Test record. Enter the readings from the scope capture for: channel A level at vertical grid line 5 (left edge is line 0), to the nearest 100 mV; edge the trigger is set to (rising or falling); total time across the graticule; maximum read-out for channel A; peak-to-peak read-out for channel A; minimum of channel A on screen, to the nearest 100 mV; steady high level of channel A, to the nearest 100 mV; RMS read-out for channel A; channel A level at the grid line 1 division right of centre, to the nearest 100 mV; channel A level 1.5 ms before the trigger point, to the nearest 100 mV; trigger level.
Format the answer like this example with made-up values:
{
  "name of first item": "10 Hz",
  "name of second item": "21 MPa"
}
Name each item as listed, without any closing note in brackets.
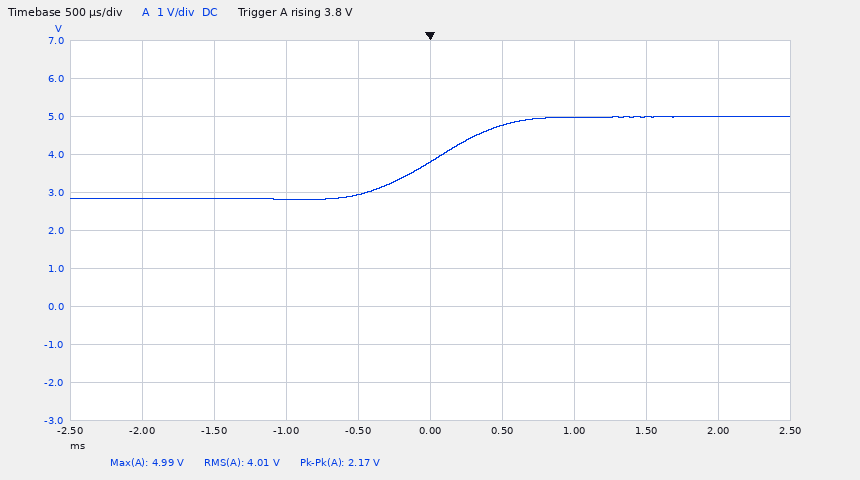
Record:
{
  "channel A level at vertical grid line 5 (left edge is line 0), to the nearest 100 mV": "3.8 V",
  "edge the trigger is set to": "rising",
  "total time across the graticule": "5 ms",
  "maximum read-out for channel A": "4.99 V",
  "peak-to-peak read-out for channel A": "2.17 V",
  "minimum of channel A on screen, to the nearest 100 mV": "2.8 V",
  "steady high level of channel A, to the nearest 100 mV": "5.0 V",
  "RMS read-out for channel A": "4.01 V",
  "channel A level at the grid line 1 division right of centre, to the nearest 100 mV": "4.8 V",
  "channel A level 1.5 ms before the trigger point, to the nearest 100 mV": "2.8 V",
  "trigger level": "3.8 V"
}
